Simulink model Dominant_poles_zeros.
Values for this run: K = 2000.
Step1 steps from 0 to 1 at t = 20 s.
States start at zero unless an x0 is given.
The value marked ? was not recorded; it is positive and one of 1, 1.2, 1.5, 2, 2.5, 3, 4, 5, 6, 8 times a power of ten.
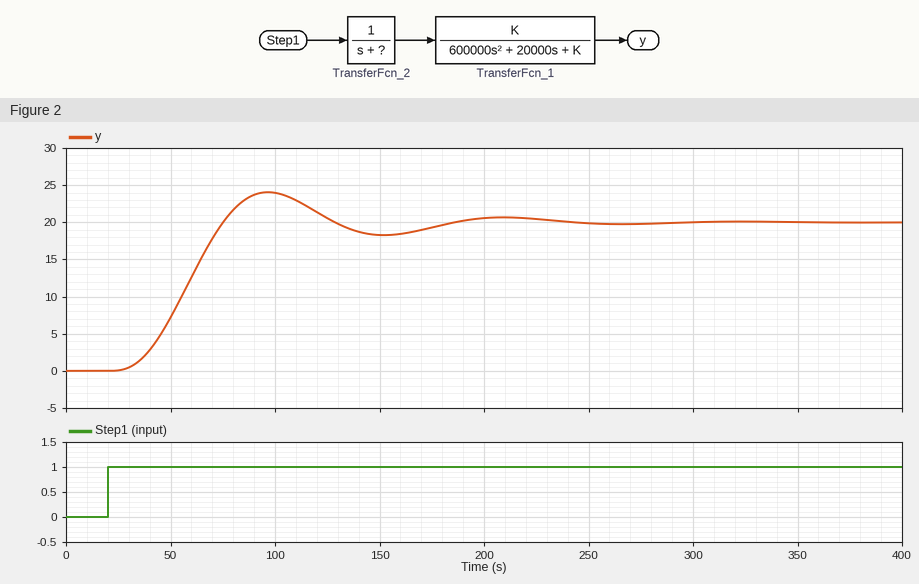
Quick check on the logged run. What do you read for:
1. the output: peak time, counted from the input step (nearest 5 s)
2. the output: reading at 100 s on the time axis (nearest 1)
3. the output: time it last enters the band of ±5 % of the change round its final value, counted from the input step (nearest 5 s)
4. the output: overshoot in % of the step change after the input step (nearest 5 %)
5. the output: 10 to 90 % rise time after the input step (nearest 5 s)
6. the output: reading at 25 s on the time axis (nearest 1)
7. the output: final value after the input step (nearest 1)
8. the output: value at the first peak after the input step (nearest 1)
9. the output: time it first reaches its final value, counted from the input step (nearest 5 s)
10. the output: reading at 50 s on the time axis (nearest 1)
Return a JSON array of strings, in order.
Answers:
["75 s", "24", "150 s", "20 %", "35 s", "0", "20", "24", "55 s", "7"]
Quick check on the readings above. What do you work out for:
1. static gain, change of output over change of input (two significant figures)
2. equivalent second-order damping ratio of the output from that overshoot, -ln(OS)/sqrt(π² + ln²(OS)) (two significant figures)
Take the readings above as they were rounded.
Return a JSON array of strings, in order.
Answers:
["20", "0.46"]
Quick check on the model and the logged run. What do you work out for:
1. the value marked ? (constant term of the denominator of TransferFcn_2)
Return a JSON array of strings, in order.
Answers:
["0.05"]
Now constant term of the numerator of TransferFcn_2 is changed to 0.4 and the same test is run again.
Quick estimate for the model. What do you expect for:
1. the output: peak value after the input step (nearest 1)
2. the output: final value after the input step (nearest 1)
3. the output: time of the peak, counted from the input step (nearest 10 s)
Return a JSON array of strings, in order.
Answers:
["10", "8", "80 s"]
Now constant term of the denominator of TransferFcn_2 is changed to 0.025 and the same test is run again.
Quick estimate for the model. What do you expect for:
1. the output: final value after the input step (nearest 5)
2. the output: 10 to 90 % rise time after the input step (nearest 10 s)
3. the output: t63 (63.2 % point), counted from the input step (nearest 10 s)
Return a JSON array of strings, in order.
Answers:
["40", "50 s", "50 s"]
